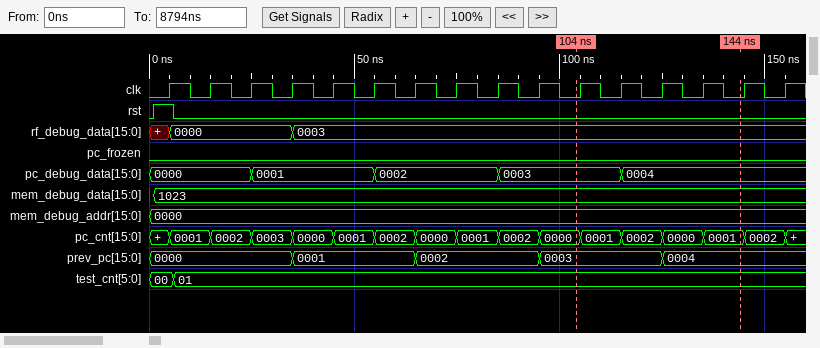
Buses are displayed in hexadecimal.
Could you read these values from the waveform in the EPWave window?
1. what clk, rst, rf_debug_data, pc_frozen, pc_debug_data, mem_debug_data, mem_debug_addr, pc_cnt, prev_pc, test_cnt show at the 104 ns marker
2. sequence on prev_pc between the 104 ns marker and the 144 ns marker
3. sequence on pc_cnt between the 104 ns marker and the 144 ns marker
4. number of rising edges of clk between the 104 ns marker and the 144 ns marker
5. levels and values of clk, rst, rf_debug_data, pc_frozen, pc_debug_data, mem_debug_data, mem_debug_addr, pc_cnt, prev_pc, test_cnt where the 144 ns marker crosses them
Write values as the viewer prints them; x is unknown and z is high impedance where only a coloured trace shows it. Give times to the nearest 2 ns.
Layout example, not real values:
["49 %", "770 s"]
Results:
["clk=0, rst=0, rf_debug_data=0003, pc_frozen=0, pc_debug_data=0003, mem_debug_data=1023, mem_debug_addr=0000, pc_cnt=0000, prev_pc=0003, test_cnt=01", "0003, 0004", "0000, 0001, 0002, 0000, 0001", "4", "clk=0, rst=0, rf_debug_data=0003, pc_frozen=0, pc_debug_data=0004, mem_debug_data=1023, mem_debug_addr=0000, pc_cnt=0001, prev_pc=0004, test_cnt=01"]
